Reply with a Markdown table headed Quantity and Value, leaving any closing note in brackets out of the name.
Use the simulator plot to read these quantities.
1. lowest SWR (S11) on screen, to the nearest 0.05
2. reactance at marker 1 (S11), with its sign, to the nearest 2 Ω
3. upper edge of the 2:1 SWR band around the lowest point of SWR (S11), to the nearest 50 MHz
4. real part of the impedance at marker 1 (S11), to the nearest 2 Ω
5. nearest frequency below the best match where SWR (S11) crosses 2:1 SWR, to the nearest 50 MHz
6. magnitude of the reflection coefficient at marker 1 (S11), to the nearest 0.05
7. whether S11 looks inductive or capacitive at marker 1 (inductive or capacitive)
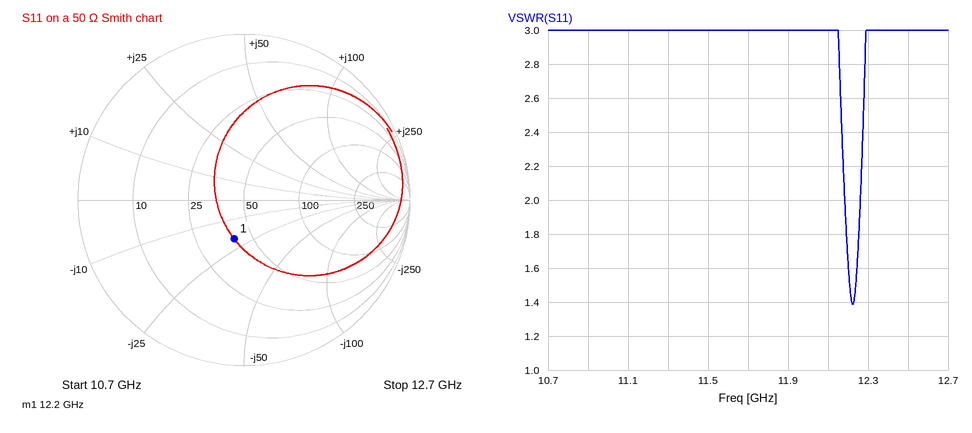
| Quantity | Value |
|---|---|
| lowest SWR (S11) on screen, to the nearest 0.05 | 1.40 |
| reactance at marker 1 (S11), with its sign, to the nearest 2 Ω | -20 Ω |
| upper edge of the 2:1 SWR band around the lowest point of SWR (S11), to the nearest 50 MHz | 12.25 GHz |
| real part of the impedance at marker 1 (S11), to the nearest 2 Ω | 40 Ω |
| nearest frequency below the best match where SWR (S11) crosses 2:1 SWR, to the nearest 50 MHz | 12.20 GHz |
| magnitude of the reflection coefficient at marker 1 (S11), to the nearest 0.05 | 0.25 |
| whether S11 looks inductive or capacitive at marker 1 | capacitive |
